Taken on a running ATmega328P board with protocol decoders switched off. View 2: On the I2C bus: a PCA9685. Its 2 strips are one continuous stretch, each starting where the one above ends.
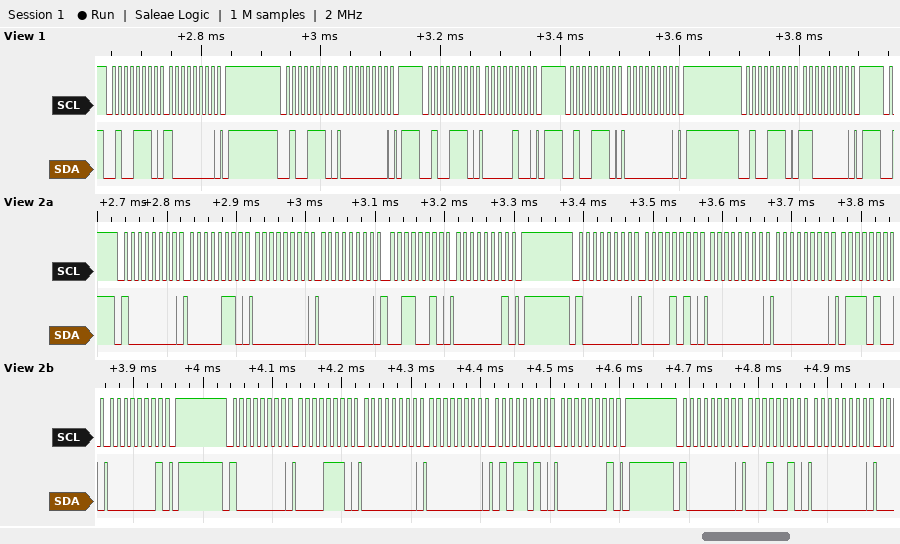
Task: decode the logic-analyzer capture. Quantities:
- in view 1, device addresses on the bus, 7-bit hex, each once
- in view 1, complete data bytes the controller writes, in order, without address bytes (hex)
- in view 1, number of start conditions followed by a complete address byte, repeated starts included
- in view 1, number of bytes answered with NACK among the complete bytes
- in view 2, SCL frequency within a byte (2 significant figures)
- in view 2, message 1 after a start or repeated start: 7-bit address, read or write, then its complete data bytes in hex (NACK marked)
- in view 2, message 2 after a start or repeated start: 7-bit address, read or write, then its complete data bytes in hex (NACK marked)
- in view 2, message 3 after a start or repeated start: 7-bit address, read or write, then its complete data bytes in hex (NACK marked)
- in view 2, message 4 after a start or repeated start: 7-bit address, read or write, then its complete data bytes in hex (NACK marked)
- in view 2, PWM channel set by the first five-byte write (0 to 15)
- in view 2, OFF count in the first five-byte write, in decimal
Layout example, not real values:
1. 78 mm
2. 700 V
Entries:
1. 0x27
2. 80 00 04 00 C0
3. 5
4. 0
5. 100 kHz
6. 0x40 write: 06 00 00 32 01
7. 0x40 write: 0A 00 00 74 01
8. 0x40 write: 0E 00 00 5A 01
9. 0x40 write: 12 00
10. 0
11. 306
